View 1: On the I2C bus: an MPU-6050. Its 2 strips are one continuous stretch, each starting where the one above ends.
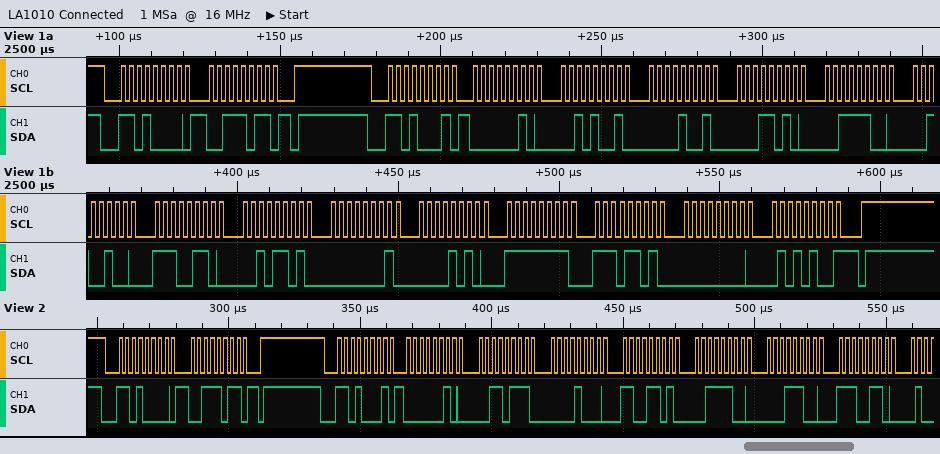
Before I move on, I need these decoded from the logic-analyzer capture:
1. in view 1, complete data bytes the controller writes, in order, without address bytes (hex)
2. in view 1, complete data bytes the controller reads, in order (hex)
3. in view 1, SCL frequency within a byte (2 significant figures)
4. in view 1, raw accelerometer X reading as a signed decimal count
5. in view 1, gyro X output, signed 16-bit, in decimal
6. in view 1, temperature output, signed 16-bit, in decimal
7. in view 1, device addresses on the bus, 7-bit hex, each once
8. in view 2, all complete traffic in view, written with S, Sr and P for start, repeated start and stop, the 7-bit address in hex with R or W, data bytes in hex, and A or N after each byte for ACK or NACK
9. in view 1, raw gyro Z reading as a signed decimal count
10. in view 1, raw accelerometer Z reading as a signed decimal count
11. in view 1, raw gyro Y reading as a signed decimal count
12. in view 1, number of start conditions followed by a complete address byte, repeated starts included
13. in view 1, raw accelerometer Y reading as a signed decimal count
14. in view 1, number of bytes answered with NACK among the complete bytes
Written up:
3B
02 29 09 1A 3C 24 E6 2D 01 0A FF ED 00 54
400 kHz
553
266
-6611
0x68
S 68W A 3B A P S 68R A 02 A 37 A 08 A CD A 3C A 1C A E6 A
84
15396
-19
2
2330
1
